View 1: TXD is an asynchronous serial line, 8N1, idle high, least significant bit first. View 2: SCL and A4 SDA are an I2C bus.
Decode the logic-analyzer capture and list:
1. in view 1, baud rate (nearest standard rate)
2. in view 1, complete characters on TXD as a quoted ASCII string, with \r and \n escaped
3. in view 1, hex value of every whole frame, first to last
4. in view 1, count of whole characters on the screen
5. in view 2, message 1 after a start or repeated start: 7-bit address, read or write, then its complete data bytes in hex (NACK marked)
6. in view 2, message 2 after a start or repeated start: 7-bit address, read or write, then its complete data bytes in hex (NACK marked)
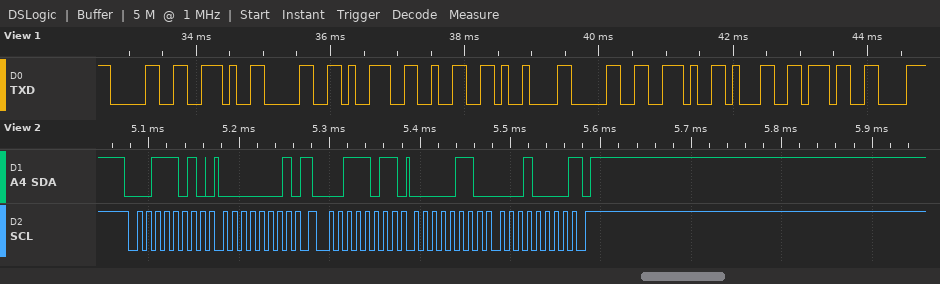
9600 baud
"0.092\t0.17"
30 2E 30 39 32 09 30 2E 31 37
10
0x1D write: 01
0x1D read: 06 10 NACK
